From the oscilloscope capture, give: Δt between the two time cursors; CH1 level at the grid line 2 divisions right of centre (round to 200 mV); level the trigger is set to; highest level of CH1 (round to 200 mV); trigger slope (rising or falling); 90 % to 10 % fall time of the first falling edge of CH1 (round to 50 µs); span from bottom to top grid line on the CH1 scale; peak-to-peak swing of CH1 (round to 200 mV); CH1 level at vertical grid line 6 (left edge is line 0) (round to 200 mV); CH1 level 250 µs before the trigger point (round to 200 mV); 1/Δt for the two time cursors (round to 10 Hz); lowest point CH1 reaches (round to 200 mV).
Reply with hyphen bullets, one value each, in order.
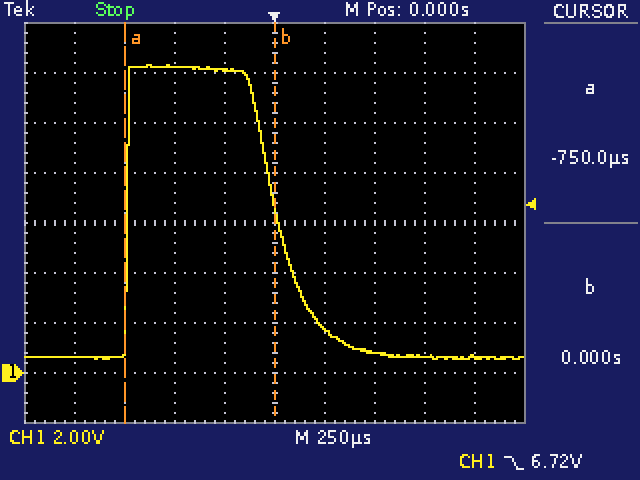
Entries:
- 750 µs
- 800 mV
- 6.72 V
- 12.4 V
- falling
- 350 µs
- 16 V
- 11.8 V
- 1.8 V
- 12.2 V
- 1.33 kHz
- 600 mV
